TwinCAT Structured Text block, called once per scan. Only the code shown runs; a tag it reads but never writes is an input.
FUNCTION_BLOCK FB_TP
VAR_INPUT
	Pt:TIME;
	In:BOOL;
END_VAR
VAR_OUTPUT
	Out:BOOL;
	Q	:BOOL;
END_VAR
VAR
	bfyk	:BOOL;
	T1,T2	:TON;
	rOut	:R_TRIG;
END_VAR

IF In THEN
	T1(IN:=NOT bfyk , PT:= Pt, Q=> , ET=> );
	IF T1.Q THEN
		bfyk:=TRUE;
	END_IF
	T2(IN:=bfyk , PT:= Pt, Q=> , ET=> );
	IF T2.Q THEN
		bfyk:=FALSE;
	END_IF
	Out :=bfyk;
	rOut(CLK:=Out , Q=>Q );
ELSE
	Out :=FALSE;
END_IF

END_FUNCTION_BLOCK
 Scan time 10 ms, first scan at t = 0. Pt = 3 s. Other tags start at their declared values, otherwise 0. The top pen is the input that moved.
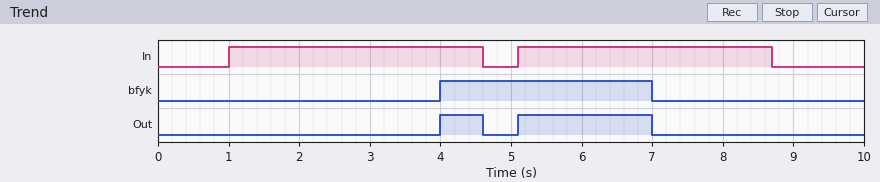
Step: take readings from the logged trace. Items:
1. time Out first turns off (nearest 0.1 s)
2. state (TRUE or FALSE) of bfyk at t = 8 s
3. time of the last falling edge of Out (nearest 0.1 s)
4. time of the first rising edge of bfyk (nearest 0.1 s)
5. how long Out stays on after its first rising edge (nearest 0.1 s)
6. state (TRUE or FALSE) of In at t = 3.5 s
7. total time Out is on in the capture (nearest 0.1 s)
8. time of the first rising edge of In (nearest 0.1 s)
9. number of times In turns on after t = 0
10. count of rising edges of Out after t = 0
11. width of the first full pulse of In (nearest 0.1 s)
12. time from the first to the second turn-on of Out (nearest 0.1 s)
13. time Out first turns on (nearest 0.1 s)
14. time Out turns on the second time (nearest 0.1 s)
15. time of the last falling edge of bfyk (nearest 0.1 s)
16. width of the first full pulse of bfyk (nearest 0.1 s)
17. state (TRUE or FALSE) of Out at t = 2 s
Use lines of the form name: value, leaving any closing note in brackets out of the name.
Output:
time Out first turns off: 4.6 s
state (TRUE or FALSE) of bfyk at t = 8 s: FALSE
time of the last falling edge of Out: 7.0 s
time of the first rising edge of bfyk: 4.0 s
how long Out stays on after its first rising edge: 0.6 s
state (TRUE or FALSE) of In at t = 3.5 s: TRUE
total time Out is on in the capture: 2.5 s
time of the first rising edge of In: 1.0 s
number of times In turns on after t = 0: 2
count of rising edges of Out after t = 0: 2
width of the first full pulse of In: 3.6 s
time from the first to the second turn-on of Out: 1.1 s
time Out first turns on: 4.0 s
time Out turns on the second time: 5.1 s
time of the last falling edge of bfyk: 7.0 s
width of the first full pulse of bfyk: 3.0 s
state (TRUE or FALSE) of Out at t = 2 s: FALSE
